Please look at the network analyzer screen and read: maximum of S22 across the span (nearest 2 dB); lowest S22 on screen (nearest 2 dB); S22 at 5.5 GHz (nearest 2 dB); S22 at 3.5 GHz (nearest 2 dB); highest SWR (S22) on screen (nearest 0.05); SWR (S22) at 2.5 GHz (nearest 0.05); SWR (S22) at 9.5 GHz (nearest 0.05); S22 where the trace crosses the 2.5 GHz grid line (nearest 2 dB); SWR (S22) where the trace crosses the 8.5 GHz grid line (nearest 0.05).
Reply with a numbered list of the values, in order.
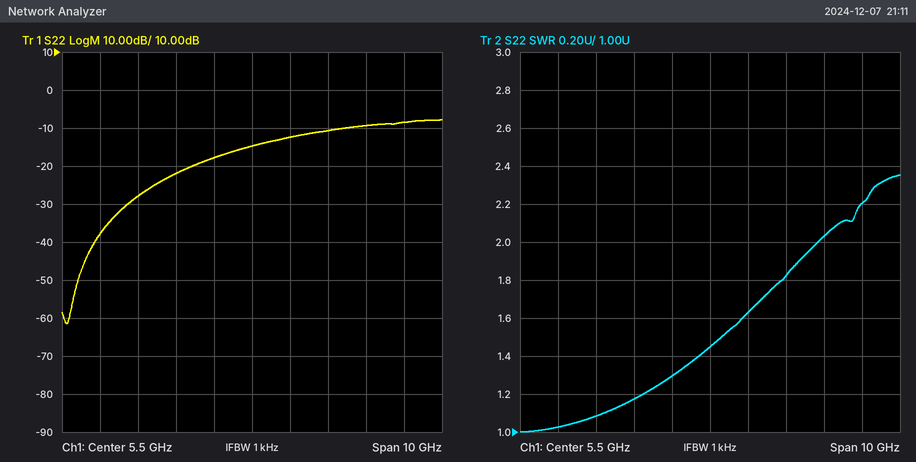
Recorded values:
1. -8 dB
2. -62 dB
3. -14 dB
4. -22 dB
5. 2.35
6. 1.10
7. 2.20
8. -28 dB
9. 2.05
